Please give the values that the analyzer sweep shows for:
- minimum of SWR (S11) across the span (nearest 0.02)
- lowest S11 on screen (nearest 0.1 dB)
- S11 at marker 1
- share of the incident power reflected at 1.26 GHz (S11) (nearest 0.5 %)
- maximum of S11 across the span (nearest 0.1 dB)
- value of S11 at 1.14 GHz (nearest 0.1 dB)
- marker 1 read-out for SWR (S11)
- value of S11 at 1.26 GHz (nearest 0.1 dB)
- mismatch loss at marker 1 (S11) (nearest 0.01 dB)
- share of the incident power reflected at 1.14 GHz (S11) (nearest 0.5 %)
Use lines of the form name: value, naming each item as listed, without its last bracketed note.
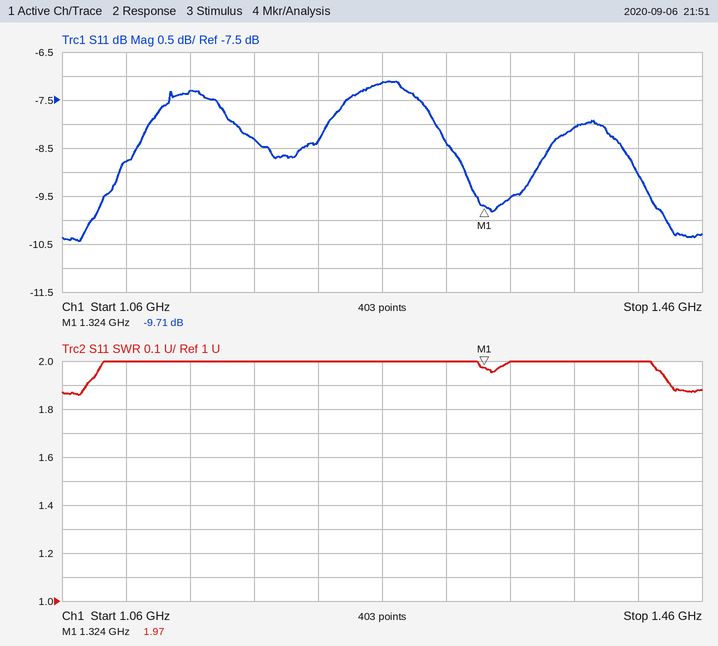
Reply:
minimum of SWR (S11) across the span: 1.86
lowest S11 on screen: -10.4 dB
S11 at marker 1: -9.71 dB
share of the incident power reflected at 1.26 GHz (S11): 19.5 %
maximum of S11 across the span: -7.1 dB
value of S11 at 1.14 GHz: -7.3 dB
marker 1 read-out for SWR: 1.97
value of S11 at 1.26 GHz: -7.1 dB
mismatch loss at marker 1 (S11): 0.49 dB
share of the incident power reflected at 1.14 GHz (S11): 18.5 %
